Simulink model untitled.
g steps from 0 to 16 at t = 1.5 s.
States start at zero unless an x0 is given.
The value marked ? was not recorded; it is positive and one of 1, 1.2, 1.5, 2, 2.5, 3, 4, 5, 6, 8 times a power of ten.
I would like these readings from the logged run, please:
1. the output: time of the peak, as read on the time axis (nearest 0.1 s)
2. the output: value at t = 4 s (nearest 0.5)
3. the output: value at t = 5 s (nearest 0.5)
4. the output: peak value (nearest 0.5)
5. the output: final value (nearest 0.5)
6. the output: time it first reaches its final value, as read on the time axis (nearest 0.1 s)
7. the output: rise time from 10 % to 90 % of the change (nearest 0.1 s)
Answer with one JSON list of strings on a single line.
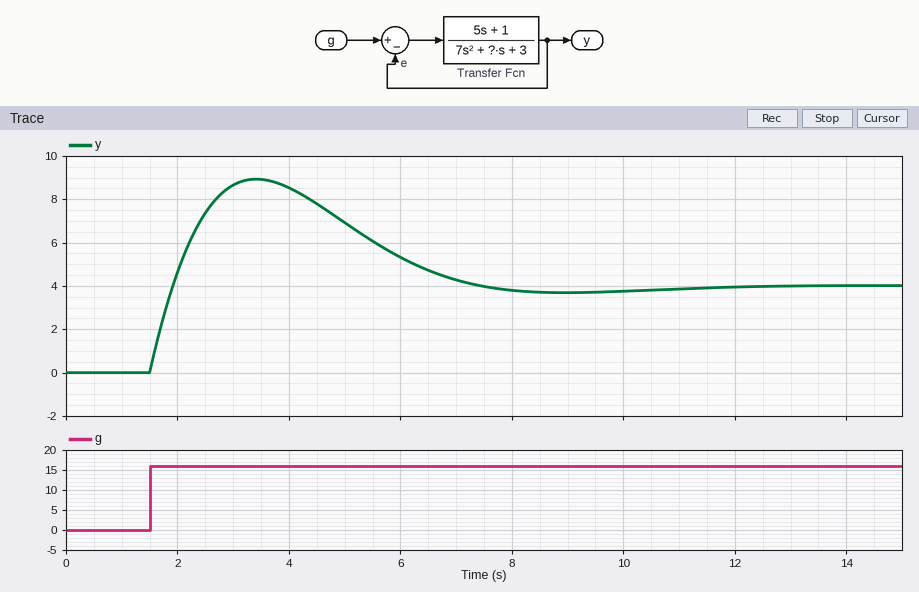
["3.4 s", "8.5", "7.0", "9.0", "4.0", "1.9 s", "0.3 s"]
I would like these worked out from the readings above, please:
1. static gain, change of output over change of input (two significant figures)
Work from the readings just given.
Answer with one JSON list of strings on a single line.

["0.25"]
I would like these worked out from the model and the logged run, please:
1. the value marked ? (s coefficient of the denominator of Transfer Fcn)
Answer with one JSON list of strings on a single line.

["2"]
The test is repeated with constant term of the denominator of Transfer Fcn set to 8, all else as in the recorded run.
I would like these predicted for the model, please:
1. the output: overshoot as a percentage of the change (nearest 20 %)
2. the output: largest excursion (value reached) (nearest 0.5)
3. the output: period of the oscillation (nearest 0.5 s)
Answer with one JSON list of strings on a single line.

["280 %", "7.0", "6.0 s"]
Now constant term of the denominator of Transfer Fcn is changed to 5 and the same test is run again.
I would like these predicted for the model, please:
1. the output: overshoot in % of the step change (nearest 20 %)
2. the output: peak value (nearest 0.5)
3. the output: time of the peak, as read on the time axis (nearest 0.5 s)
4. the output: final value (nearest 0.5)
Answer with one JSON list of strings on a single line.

["200 %", "8.0", "3.0 s", "2.5"]
